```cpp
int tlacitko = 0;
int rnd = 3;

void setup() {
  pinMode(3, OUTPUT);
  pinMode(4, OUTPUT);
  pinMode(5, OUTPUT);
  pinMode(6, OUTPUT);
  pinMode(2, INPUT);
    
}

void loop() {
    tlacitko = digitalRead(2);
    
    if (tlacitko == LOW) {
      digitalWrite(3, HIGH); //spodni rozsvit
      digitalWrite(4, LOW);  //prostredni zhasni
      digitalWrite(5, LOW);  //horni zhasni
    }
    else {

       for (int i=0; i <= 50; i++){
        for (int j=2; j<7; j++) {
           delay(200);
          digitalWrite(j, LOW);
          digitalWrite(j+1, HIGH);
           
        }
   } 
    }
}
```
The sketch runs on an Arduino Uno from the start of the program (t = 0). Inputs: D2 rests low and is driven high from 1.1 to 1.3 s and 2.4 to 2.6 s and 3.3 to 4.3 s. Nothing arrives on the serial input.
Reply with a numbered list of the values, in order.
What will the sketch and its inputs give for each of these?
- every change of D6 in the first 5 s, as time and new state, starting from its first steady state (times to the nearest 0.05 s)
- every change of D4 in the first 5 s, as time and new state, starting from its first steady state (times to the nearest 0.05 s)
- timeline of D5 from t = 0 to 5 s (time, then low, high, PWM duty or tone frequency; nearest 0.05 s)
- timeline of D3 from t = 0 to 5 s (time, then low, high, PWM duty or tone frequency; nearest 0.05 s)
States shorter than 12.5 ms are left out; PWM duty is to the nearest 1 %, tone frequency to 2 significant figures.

1. 0 s low; 1.9 s high; 2.1 s low; 2.9 s high; 3.1 s low; 3.9 s high; 4.1 s low; 4.9 s high
2. 0 s low; 1.5 s high; 1.7 s low; 2.5 s high; 2.7 s low; 3.5 s high; 3.7 s low; 4.5 s high; 4.7 s low
3. 0 s low; 1.7 s high; 1.9 s low; 2.7 s high; 2.9 s low; 3.7 s high; 3.9 s low; 4.7 s high; 4.9 s low
4. 0 s high; 1.5 s low; 2.3 s high; 2.5 s low; 3.3 s high; 3.5 s low; 4.3 s high; 4.5 s low
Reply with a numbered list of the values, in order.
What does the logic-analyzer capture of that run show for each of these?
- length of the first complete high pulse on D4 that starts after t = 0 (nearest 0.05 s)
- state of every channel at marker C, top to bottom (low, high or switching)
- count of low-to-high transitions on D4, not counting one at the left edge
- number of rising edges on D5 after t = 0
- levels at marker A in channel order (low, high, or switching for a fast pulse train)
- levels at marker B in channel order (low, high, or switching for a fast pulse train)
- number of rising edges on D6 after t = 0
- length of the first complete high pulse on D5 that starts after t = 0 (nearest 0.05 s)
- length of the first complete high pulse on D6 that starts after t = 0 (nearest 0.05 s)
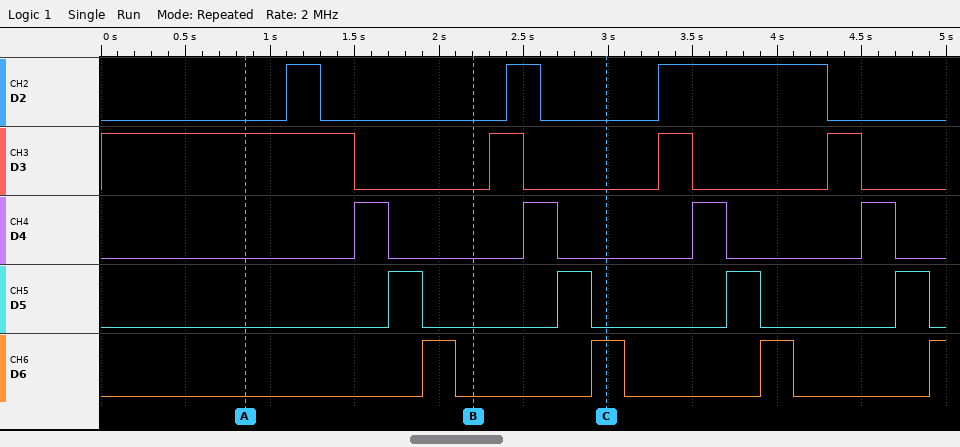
1. 0.20 s
2. D2 low, D3 low, D4 low, D5 low, D6 high
3. 4
4. 4
5. D2 low, D3 high, D4 low, D5 low, D6 low
6. D2 low, D3 low, D4 low, D5 low, D6 low
7. 4
8. 0.20 s
9. 0.20 s
